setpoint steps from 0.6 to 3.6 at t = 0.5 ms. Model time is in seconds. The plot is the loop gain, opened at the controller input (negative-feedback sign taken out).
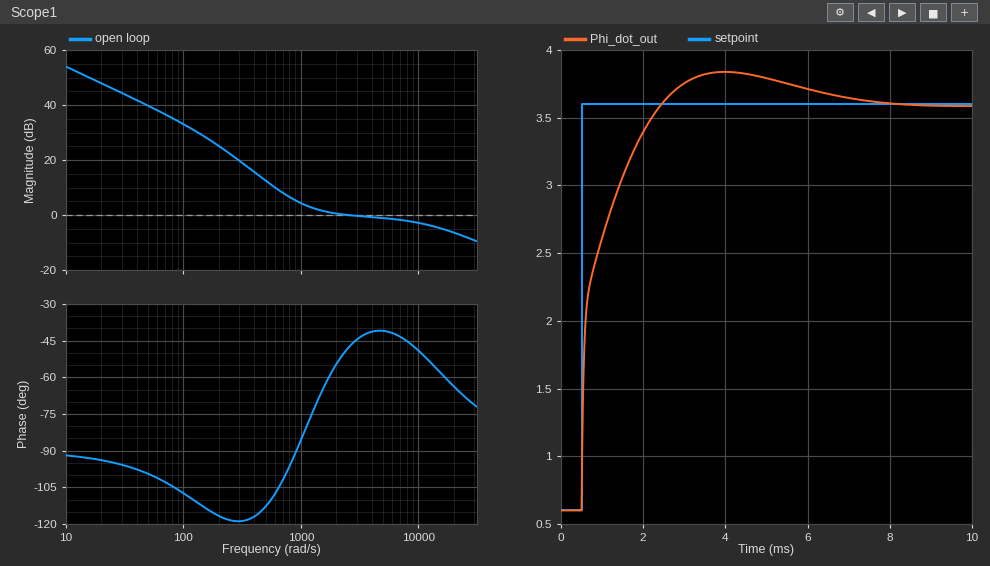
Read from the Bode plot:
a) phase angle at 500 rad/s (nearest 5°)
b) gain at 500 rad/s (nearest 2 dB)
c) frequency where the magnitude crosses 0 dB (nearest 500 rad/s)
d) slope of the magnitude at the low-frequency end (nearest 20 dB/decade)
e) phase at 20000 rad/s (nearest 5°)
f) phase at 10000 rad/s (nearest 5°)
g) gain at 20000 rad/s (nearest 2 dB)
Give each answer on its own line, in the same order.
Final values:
-115°
12 dB
2500 rad/s
-20 dB/decade
-65°
-50°
-6 dB
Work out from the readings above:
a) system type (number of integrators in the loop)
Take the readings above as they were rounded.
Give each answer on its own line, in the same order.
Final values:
1
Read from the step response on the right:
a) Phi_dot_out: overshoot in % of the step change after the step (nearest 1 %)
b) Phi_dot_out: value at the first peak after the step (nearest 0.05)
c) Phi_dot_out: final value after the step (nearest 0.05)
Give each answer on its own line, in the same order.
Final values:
8 %
3.85
3.60
